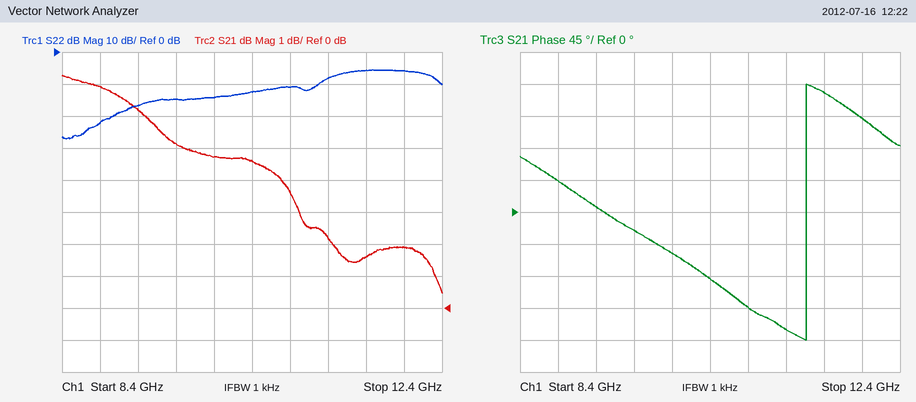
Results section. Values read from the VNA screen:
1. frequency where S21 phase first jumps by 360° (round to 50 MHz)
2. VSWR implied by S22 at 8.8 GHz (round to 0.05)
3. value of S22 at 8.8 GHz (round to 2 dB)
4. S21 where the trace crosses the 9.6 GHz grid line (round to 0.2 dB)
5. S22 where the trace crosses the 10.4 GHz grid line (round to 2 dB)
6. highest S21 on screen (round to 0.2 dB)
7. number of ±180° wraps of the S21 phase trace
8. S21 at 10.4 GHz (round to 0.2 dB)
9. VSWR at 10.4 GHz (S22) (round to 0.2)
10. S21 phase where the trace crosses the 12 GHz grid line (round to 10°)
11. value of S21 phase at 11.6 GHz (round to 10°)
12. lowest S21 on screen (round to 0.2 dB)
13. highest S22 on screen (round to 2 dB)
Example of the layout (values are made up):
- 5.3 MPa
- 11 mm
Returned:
- 11.40 GHz
- 1.15
- -22 dB
- 5.2 dB
- -12 dB
- 7.2 dB
- 1
- 4.6 dB
- 1.6
- 130°
- 170°
- 0.4 dB
- -6 dB
